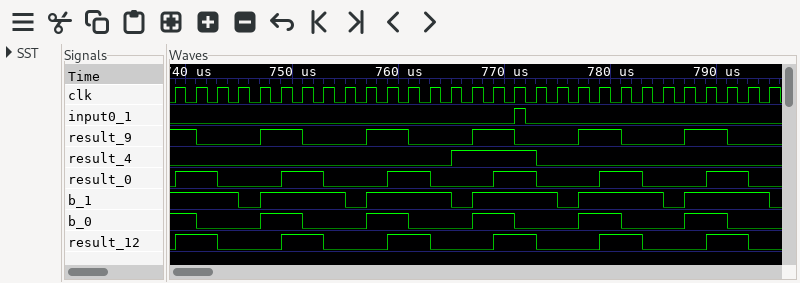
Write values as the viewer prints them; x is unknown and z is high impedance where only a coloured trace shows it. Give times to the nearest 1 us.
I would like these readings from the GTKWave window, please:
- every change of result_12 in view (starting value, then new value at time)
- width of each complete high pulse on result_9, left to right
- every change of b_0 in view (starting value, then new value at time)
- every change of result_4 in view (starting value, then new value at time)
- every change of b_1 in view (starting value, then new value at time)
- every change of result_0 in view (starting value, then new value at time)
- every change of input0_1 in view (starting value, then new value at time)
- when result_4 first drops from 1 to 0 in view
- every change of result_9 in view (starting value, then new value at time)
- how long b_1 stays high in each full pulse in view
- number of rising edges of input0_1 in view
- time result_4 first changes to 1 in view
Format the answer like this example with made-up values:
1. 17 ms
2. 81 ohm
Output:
1. 0, 1 at 739 us, 0 at 743 us, 1 at 749 us, 0 at 753 us, 1 at 759 us, 0 at 763 us, 1 at 769 us, 0 at 773 us, 1 at 779 us, 0 at 783 us, 1 at 789 us, 0 at 793 us
2. 4 us, 4 us, 4 us, 4 us, 4 us
3. 1, 0 at 741 us, 1 at 747 us, 0 at 751 us, 1 at 757 us, 0 at 761 us, 1 at 767 us, 0 at 771 us, 1 at 777 us, 0 at 781 us, 1 at 787 us, 0 at 791 us
4. 0, 1 at 765 us, 0 at 773 us
5. 1, 0 at 745 us, 1 at 747 us, 0 at 755 us, 1 at 757 us, 0 at 765 us, 1 at 767 us, 0 at 775 us, 1 at 777 us, 0 at 785 us, 1 at 787 us, 0 at 795 us
6. 0, 1 at 739 us, 0 at 743 us, 1 at 749 us, 0 at 753 us, 1 at 759 us, 0 at 763 us, 1 at 769 us, 0 at 773 us, 1 at 779 us, 0 at 783 us, 1 at 789 us, 0 at 793 us
7. 0, 1 at 771 us, 0 at 772 us
8. 773 us
9. 1, 0 at 741 us, 1 at 747 us, 0 at 751 us, 1 at 757 us, 0 at 761 us, 1 at 767 us, 0 at 771 us, 1 at 777 us, 0 at 781 us, 1 at 787 us, 0 at 791 us
10. 8 us, 8 us, 8 us, 8 us, 8 us
11. 1
12. 765 us
